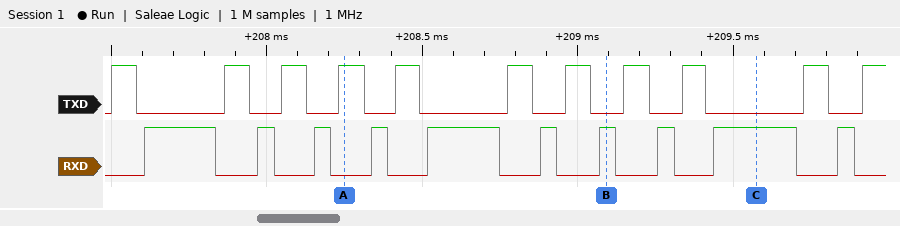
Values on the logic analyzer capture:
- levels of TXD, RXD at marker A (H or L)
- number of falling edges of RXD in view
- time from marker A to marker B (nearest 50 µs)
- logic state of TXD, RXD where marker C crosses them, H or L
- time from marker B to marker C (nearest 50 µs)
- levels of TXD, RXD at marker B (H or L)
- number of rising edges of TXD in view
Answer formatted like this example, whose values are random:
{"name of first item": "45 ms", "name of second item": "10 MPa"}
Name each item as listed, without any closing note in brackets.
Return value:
{"levels of TXD, RXD at marker A": "TXD=H, RXD=L", "number of falling edges of RXD in view": "10", "time from marker A to marker B": "850 µs", "logic state of TXD, RXD where marker C crosses them, H or L": "TXD=L, RXD=H", "time from marker B to marker C": "500 µs", "levels of TXD, RXD at marker B": "TXD=L, RXD=H", "number of rising edges of TXD in view": "11"}
